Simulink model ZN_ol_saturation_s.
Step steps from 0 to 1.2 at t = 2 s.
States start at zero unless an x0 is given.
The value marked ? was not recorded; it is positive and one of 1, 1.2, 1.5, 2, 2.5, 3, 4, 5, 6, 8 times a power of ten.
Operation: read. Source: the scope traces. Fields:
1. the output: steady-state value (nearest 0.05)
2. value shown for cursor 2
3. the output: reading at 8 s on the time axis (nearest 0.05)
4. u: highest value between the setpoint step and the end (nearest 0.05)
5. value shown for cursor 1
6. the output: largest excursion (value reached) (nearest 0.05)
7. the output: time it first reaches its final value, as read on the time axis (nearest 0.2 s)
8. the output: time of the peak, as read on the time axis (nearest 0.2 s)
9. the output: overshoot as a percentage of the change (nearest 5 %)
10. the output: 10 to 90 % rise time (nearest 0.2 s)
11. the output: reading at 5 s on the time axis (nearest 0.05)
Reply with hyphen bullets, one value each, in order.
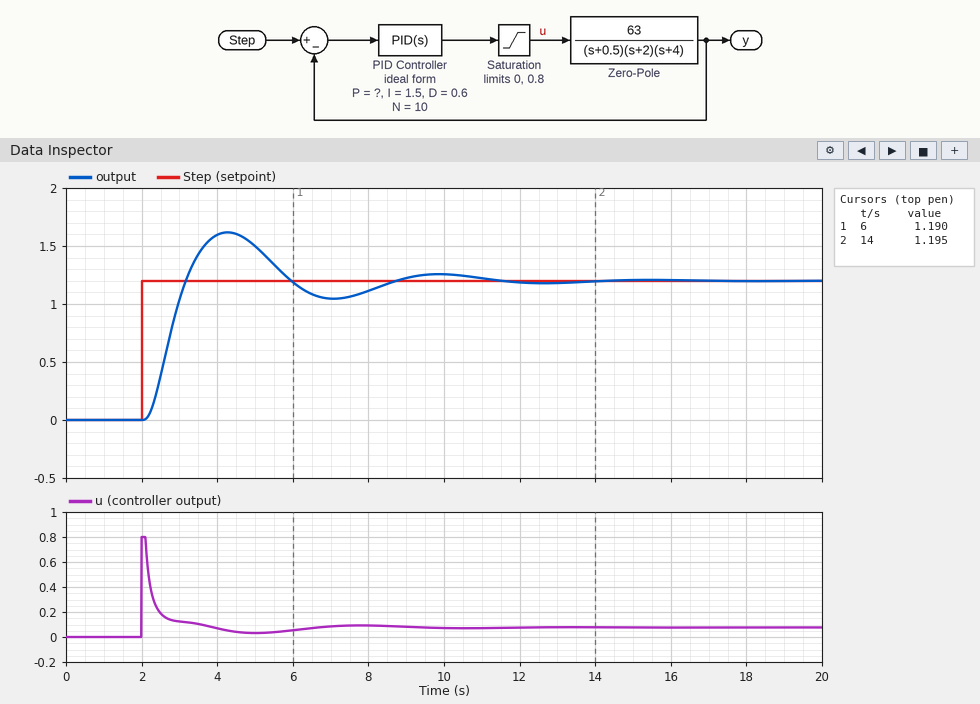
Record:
- 1.20
- 1.195
- 1.10
- 0.80
- 1.190
- 1.60
- 3.2 s
- 4.2 s
- 35 %
- 0.8 s
- 1.50
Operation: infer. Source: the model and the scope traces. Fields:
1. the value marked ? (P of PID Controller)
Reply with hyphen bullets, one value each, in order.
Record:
- 0.2
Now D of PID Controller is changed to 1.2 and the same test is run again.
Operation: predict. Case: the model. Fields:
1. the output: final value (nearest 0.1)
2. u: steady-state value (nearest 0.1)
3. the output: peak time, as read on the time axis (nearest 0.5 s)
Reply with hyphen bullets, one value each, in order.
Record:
- 1.2
- 0.1
- 5.0 s
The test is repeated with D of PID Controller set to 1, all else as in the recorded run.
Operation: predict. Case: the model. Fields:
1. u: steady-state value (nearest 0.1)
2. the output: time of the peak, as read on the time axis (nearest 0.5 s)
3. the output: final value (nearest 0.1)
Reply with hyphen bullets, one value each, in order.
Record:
- 0.1
- 5.0 s
- 1.2
